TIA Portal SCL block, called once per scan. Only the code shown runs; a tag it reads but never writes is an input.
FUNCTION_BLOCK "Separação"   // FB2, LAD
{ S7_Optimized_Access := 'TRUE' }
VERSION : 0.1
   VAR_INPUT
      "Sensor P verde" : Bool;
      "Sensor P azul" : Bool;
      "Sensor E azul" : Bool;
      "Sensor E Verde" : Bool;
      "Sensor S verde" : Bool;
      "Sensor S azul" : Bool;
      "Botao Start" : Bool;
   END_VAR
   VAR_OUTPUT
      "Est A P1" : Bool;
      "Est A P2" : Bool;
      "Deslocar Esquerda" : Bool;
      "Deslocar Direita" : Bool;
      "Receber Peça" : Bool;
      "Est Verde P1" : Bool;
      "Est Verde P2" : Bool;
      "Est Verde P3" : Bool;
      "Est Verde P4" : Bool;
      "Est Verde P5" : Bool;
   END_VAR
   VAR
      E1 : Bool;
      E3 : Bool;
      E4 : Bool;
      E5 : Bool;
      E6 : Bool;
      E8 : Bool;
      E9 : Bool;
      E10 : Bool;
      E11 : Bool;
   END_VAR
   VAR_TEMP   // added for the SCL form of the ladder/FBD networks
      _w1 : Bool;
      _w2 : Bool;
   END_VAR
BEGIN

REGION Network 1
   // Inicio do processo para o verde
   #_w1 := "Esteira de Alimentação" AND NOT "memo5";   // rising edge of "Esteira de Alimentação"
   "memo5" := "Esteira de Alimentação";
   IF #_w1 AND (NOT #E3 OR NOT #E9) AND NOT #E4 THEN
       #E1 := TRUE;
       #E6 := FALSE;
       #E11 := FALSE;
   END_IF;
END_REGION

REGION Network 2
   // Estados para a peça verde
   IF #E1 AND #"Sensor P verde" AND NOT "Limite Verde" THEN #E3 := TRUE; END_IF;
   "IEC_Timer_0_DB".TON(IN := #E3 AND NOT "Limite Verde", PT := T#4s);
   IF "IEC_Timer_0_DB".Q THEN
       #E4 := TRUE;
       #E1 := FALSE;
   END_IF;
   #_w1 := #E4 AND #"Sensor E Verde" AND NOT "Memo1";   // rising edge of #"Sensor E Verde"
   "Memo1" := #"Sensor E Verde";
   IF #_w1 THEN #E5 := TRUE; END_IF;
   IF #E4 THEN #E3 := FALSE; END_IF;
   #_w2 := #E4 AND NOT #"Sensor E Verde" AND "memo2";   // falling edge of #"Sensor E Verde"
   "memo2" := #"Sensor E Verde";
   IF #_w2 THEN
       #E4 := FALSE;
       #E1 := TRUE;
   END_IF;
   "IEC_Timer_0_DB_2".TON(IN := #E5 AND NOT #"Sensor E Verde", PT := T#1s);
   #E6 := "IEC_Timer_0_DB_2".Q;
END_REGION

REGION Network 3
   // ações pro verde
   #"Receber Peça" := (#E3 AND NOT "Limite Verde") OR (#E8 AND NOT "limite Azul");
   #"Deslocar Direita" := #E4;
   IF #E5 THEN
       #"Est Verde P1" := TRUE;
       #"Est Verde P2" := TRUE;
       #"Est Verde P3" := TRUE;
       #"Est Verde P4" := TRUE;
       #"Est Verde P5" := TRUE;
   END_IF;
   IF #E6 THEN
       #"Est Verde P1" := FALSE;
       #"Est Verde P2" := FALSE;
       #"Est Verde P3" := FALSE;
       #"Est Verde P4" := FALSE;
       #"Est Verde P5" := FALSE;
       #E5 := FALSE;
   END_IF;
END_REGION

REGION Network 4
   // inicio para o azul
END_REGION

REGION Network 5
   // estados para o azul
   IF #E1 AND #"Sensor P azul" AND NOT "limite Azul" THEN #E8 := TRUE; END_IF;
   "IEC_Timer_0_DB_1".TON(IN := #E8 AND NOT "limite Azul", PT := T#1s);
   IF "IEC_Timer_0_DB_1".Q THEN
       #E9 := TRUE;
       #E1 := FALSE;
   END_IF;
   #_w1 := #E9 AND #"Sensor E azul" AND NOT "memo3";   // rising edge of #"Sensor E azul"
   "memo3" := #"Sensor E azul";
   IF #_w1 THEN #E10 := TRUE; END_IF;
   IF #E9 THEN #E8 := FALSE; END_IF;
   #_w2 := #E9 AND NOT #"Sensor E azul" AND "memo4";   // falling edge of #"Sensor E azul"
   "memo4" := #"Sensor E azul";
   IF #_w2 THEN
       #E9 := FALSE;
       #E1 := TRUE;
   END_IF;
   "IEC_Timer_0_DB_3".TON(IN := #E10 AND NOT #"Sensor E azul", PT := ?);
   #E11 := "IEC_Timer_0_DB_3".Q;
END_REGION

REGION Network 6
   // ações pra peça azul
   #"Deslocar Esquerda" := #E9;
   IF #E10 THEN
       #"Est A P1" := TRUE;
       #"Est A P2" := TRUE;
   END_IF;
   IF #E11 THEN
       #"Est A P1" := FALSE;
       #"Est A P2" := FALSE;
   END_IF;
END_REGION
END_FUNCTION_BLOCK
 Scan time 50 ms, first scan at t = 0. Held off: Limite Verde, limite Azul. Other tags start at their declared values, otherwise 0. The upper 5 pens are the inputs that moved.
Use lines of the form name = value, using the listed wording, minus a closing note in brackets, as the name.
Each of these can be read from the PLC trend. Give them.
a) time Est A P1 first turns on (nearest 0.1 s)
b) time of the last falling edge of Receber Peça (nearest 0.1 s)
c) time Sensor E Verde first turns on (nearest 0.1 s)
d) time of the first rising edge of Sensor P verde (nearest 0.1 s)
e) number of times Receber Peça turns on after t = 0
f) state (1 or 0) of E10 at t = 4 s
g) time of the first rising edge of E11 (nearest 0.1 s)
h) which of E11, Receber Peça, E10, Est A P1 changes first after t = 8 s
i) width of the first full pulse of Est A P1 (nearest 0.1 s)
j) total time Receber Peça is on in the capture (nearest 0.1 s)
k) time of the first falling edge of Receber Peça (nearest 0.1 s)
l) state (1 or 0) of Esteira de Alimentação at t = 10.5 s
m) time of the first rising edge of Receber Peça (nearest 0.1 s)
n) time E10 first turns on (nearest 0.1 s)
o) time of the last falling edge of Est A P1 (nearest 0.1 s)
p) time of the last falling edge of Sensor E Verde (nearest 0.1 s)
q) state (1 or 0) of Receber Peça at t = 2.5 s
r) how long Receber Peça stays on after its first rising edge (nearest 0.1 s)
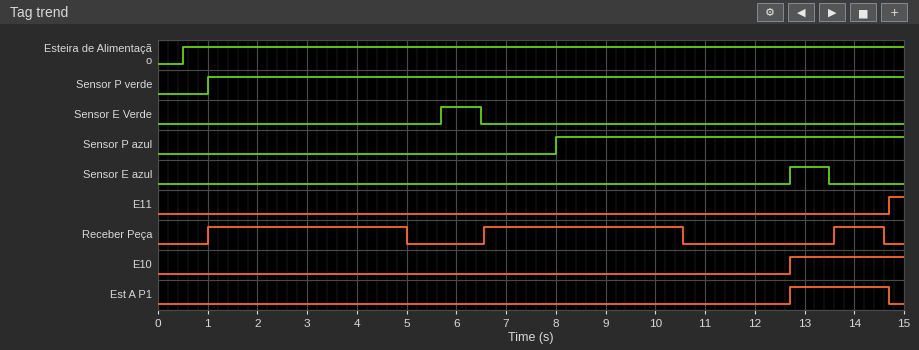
time Est A P1 first turns on = 12.7 s
time of the last falling edge of Receber Peça = 14.6 s
time Sensor E Verde first turns on = 5.7 s
time of the first rising edge of Sensor P verde = 1.0 s
number of times Receber Peça turns on after t = 0 = 3
state (1 or 0) of E10 at t = 4 s = 0
time of the first rising edge of E11 = 14.7 s
which of E11, Receber Peça, E10, Est A P1 changes first after t = 8 s = Receber Peça
width of the first full pulse of Est A P1 = 2.0 s
total time Receber Peça is on in the capture = 9.0 s
time of the first falling edge of Receber Peça = 5.0 s
state (1 or 0) of Esteira de Alimentação at t = 10.5 s = 1
time of the first rising edge of Receber Peça = 1.0 s
time E10 first turns on = 12.7 s
time of the last falling edge of Est A P1 = 14.7 s
time of the last falling edge of Sensor E Verde = 6.5 s
state (1 or 0) of Receber Peça at t = 2.5 s = 1
how long Receber Peça stays on after its first rising edge = 4.0 s
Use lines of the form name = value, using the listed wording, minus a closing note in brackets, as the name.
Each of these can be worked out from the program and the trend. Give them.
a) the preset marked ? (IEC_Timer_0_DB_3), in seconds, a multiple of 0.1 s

the preset marked ? (IEC_Timer_0_DB_3), in seconds, a multiple of 0.1 s = 1.2 s
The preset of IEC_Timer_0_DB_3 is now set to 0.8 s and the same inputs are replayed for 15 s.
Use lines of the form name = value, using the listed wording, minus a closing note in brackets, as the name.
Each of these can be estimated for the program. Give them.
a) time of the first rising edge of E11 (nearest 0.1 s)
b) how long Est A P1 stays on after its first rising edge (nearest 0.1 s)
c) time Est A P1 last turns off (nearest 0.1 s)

time of the first rising edge of E11 = 14.3 s
how long Est A P1 stays on after its first rising edge = 1.6 s
time Est A P1 last turns off = 14.3 s
